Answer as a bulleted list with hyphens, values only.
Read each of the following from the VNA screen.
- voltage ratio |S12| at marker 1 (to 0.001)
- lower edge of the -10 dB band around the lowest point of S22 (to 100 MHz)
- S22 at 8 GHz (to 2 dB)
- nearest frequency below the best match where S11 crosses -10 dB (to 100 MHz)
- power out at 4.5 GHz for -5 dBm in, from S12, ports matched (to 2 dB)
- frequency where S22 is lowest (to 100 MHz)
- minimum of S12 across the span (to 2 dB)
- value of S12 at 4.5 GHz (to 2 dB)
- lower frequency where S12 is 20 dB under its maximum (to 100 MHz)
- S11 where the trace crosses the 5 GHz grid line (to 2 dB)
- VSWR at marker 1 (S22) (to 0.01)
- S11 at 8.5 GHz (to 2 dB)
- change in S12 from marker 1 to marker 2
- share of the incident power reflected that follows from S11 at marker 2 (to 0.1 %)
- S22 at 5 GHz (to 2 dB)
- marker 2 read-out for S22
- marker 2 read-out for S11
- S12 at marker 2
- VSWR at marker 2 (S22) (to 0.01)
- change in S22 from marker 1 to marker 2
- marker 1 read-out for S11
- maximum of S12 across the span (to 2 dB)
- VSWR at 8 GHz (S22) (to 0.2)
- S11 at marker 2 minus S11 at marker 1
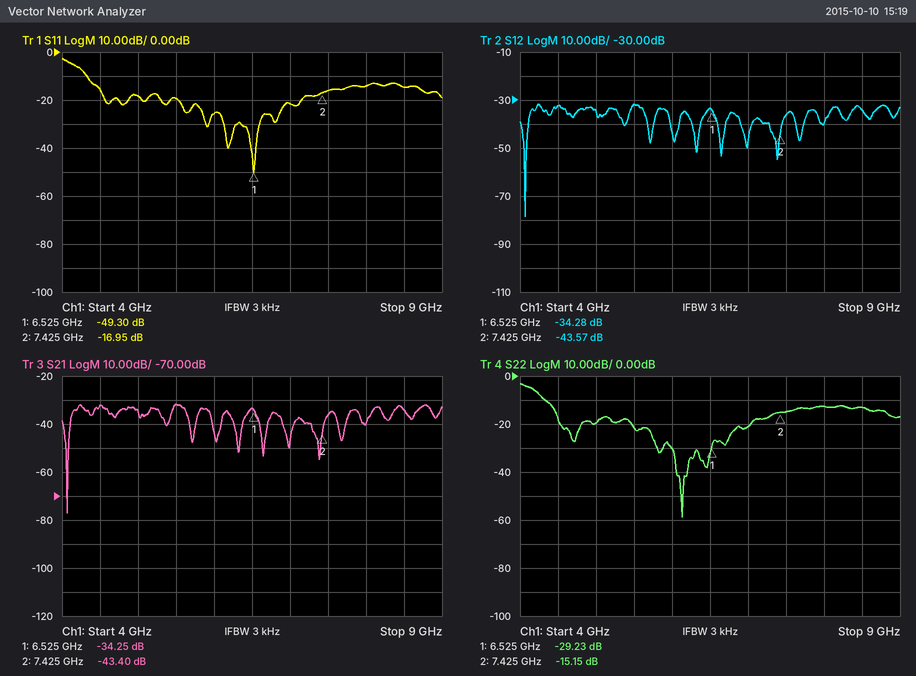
- 0.019
- 4.3 GHz
- -12 dB
- 4.3 GHz
- -38 dBm
- 6.1 GHz
- -78 dB
- -32 dB
- 4.1 GHz
- -18 dB
- 1.07
- -14 dB
- -9.29 dB
- 2.0 %
- -20 dB
- -15.15 dB
- -16.95 dB
- -43.57 dB
- 1.42
- 14.08 dB
- -49.30 dB
- -32 dB
- 1.6
- 32.35 dB
